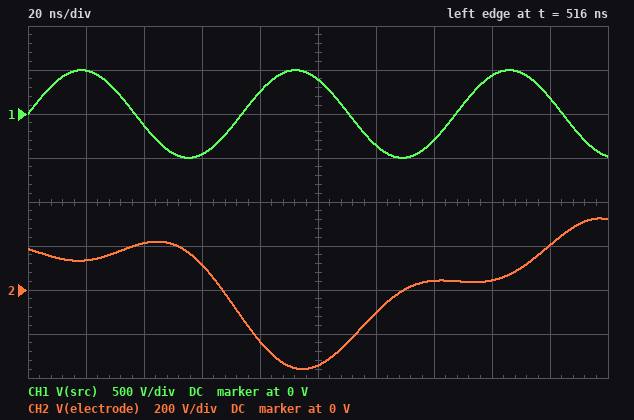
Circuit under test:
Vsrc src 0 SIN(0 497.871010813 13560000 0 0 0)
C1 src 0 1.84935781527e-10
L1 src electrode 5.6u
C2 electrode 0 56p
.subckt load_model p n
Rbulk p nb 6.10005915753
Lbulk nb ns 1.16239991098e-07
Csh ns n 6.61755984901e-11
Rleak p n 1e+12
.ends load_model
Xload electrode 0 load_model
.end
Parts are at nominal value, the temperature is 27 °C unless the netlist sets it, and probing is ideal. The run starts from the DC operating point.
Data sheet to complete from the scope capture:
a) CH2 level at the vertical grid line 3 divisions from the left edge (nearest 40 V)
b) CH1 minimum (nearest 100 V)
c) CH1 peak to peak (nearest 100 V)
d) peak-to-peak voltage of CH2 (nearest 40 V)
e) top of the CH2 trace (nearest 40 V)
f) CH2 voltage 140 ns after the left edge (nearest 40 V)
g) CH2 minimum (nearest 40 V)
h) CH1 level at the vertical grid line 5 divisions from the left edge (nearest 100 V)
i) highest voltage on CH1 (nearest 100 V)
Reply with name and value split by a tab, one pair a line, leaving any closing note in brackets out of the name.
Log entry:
CH2 level at the vertical grid line 3 divisions from the left edge	120 V
CH1 minimum	-500 V
CH1 peak to peak	1.0 kV
peak-to-peak voltage of CH2	680 V
top of the CH2 trace	320 V
CH2 voltage 140 ns after the left edge	40 V
CH2 minimum	-360 V
CH1 level at the vertical grid line 5 divisions from the left edge	400 V
highest voltage on CH1	500 V
